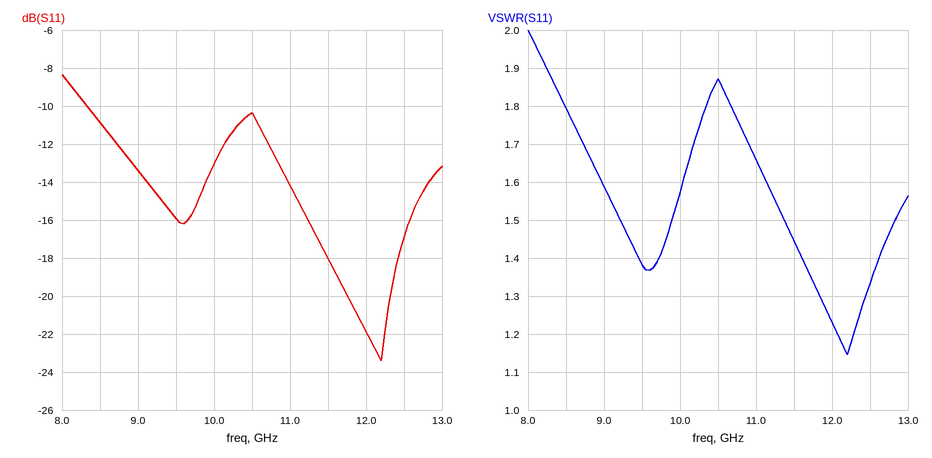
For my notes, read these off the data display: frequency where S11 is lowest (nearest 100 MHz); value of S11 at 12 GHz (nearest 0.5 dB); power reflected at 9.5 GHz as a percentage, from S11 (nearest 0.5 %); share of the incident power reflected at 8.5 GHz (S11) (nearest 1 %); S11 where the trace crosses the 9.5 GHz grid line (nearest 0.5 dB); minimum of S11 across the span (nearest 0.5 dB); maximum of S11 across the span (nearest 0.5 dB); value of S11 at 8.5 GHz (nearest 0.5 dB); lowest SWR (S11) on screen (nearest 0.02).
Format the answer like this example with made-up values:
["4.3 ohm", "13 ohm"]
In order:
["12.2 GHz", "-22.0 dB", "2.5 %", "8 %", "-16.0 dB", "-23.5 dB", "-8.5 dB", "-11.0 dB", "1.14"]
